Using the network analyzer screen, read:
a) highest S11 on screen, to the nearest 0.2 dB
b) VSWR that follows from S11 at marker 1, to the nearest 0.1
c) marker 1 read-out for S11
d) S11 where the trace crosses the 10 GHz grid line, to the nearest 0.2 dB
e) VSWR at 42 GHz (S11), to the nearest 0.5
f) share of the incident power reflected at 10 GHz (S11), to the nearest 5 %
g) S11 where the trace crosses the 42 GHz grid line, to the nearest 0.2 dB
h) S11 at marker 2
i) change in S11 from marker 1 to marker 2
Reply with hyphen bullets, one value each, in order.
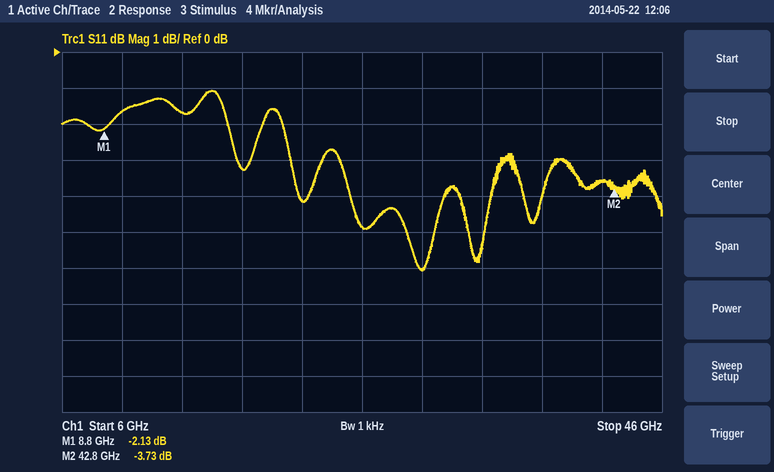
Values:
- -1.0 dB
- 8.2
- -2.13 dB
- -1.6 dB
- 5.0
- 70 %
- -3.6 dB
- -3.73 dB
- -1.60 dB
